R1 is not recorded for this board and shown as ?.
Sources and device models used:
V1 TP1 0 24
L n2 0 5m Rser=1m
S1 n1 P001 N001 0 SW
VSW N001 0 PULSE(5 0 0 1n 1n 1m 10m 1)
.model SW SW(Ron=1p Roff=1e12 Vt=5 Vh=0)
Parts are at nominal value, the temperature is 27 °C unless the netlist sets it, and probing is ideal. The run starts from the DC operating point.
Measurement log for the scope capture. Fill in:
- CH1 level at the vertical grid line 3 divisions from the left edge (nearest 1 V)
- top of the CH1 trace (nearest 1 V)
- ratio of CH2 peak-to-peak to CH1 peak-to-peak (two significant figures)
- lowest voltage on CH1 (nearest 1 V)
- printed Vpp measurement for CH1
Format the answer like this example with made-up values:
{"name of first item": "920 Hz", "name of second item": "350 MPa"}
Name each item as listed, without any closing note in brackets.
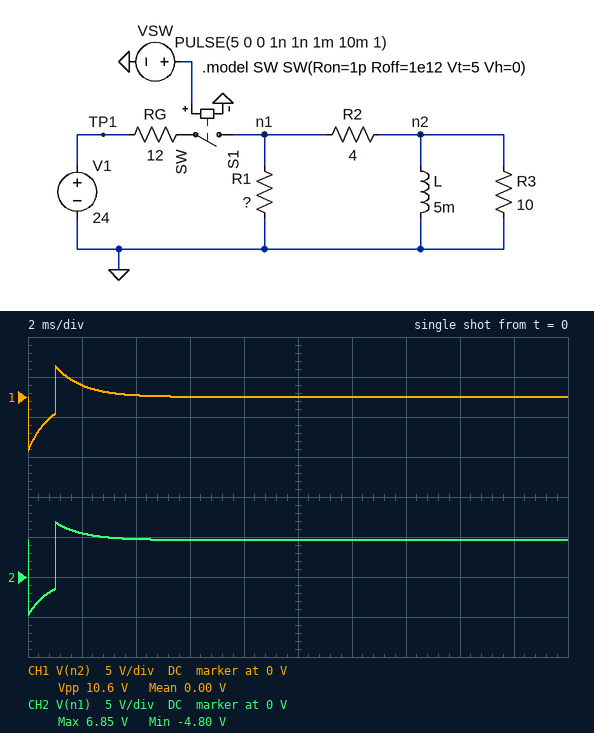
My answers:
{"CH1 level at the vertical grid line 3 divisions from the left edge": "0 V", "top of the CH1 trace": "4 V", "ratio of CH2 peak-to-peak to CH1 peak-to-peak": "1.1", "lowest voltage on CH1": "-7 V", "printed Vpp measurement for CH1": "10.6 V"}
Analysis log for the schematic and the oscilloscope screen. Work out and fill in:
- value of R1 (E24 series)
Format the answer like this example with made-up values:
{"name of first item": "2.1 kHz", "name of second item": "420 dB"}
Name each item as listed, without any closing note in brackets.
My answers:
{"value of R1": "10 Ω"}
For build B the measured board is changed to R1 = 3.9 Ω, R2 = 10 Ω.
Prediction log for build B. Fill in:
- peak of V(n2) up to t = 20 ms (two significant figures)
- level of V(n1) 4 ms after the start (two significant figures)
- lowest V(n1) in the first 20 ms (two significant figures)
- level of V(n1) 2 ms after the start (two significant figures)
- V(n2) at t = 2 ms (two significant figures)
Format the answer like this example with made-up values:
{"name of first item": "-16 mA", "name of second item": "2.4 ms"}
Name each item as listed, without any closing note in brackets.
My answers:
{"peak of V(n2) up to t = 20 ms": "1.8 V", "level of V(n1) 4 ms after the start": "4.6 V", "lowest V(n1) in the first 20 ms": "-740 mV", "level of V(n1) 2 ms after the start": "4.7 V", "V(n2) at t = 2 ms": "570 mV"}
